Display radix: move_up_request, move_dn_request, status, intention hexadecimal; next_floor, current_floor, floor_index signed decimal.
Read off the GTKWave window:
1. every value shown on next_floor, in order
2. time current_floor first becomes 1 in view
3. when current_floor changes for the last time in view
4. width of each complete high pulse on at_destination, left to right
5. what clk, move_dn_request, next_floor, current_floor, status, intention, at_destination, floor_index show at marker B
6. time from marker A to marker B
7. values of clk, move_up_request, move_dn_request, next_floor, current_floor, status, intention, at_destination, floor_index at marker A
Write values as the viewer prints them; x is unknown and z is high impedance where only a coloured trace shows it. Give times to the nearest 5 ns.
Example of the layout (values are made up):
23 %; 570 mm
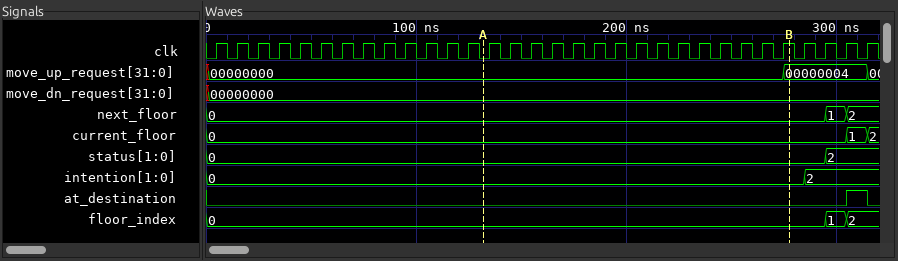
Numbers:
0, 1, 2; 305 ns; 315 ns; 10 ns; clk=1, move_dn_request=00000000, next_floor=0, current_floor=0, status=0, intention=0, at_destination=0, floor_index=0; 145 ns; clk=0, move_up_request=00000000, move_dn_request=00000000, next_floor=0, current_floor=0, status=0, intention=0, at_destination=0, floor_index=0
